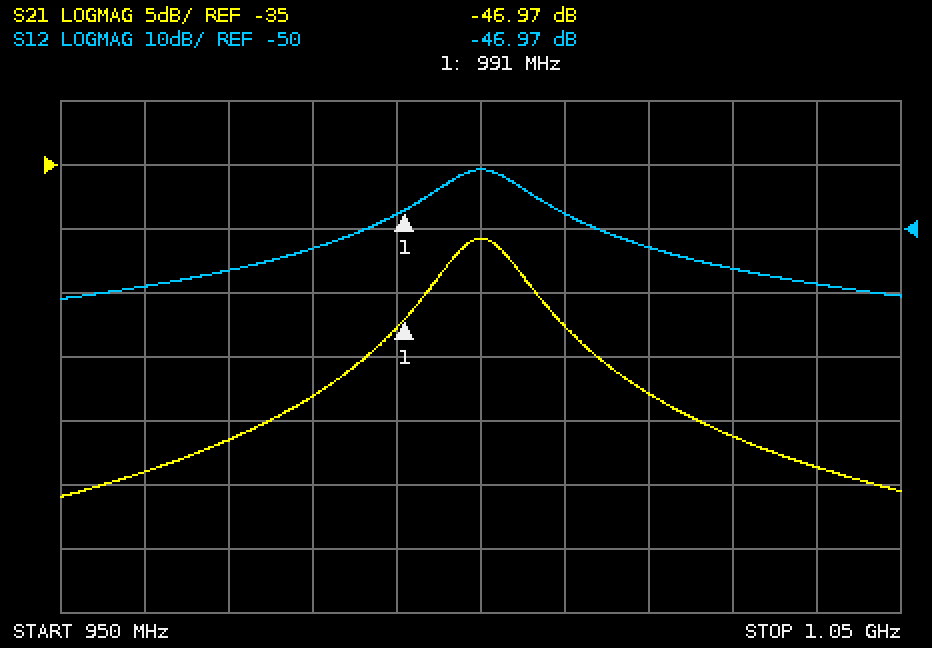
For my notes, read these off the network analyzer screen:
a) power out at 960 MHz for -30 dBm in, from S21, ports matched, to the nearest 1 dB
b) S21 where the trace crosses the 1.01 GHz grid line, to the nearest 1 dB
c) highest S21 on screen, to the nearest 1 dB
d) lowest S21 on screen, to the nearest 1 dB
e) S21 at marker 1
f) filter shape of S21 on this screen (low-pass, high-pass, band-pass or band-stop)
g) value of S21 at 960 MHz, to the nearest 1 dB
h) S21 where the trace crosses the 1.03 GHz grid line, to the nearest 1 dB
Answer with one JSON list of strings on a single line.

["-89 dBm", "-48 dB", "-41 dB", "-61 dB", "-46.97 dB", "band-pass", "-59 dB", "-56 dB"]
